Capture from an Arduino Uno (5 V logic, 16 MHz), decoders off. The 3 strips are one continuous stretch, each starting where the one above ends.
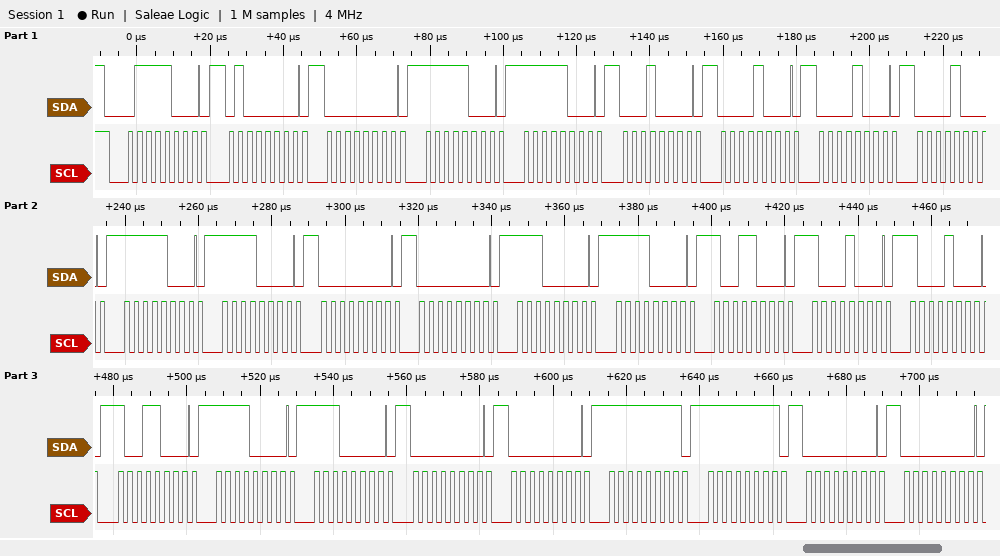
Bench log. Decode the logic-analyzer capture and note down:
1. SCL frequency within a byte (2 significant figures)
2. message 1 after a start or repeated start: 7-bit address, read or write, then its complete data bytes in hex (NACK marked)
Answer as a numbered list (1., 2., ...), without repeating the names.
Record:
1. 400 kHz
2. 0x3C write: 40 00 F8 F8 10 08 08 08 F8 F0 00 00 E0 F0 98 88 88 98 F0 E0 00 00 FF FF 00 00
